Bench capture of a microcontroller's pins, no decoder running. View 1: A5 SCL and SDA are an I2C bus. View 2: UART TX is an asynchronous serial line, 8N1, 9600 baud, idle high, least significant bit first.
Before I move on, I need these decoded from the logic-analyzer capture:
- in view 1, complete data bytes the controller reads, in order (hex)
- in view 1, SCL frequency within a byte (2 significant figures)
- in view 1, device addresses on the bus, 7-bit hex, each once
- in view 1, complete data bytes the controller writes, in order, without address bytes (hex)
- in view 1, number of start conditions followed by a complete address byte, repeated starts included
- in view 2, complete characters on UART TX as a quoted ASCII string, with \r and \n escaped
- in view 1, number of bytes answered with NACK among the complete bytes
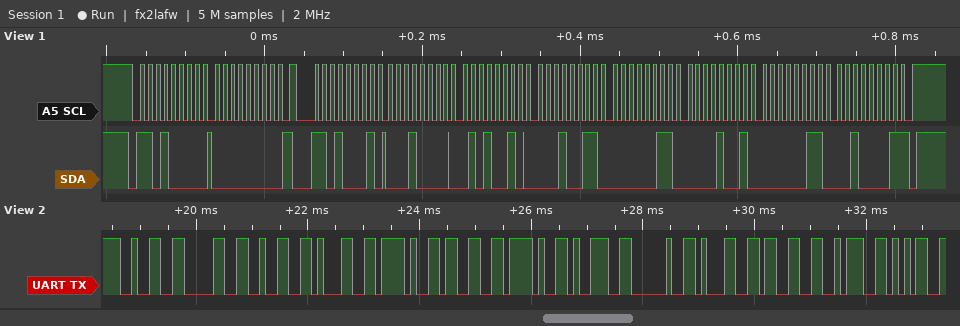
10 52 13 03 09 03 21
100 kHz
0x68
00
2
"2021/3/9 13:5"
1
